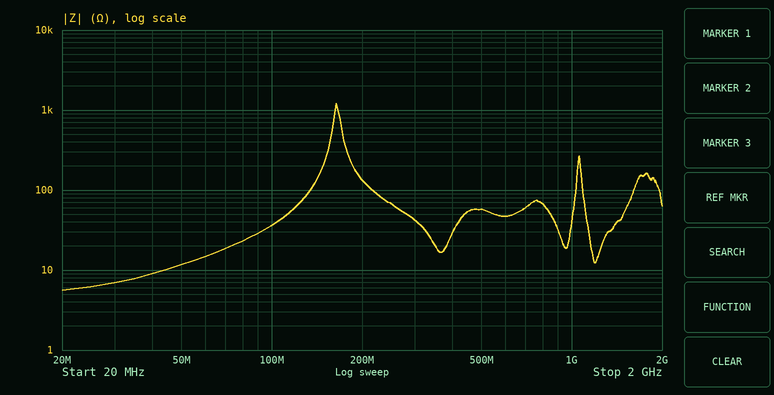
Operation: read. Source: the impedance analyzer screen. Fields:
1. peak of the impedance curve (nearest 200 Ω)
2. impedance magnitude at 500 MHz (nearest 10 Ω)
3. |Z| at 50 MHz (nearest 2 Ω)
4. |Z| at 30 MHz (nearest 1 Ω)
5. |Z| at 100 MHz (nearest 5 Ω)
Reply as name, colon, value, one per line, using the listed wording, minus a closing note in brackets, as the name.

peak of the impedance curve: 1.2 kΩ
impedance magnitude at 500 MHz: 60 Ω
|Z| at 50 MHz: 12 Ω
|Z| at 30 MHz: 7 Ω
|Z| at 100 MHz: 35 Ω
